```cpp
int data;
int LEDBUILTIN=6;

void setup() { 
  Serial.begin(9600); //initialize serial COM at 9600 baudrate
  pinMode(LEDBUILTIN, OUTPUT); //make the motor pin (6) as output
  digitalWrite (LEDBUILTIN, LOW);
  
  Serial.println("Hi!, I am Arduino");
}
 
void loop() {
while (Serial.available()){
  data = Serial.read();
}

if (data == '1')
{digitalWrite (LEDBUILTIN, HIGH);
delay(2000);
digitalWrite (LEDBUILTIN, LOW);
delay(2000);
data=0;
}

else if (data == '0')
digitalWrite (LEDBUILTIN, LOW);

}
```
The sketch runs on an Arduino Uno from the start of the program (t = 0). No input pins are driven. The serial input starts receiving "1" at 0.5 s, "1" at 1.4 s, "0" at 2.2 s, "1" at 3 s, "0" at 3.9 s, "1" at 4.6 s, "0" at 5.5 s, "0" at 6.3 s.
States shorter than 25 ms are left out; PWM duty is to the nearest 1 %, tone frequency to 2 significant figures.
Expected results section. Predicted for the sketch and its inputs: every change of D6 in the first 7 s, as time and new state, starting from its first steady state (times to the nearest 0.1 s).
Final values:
0 s low; 0.5 s high; 2.5 s low; 4.6 s high; 6.6 s low
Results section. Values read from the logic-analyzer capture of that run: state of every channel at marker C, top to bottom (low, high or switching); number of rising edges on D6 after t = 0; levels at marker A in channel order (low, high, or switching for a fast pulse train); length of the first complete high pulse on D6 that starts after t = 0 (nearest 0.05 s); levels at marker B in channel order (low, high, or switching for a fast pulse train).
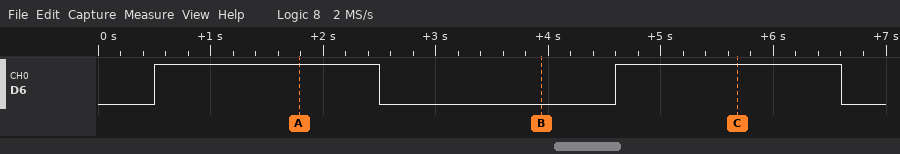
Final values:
D6 high
2
D6 high
2.00 s
D6 low
